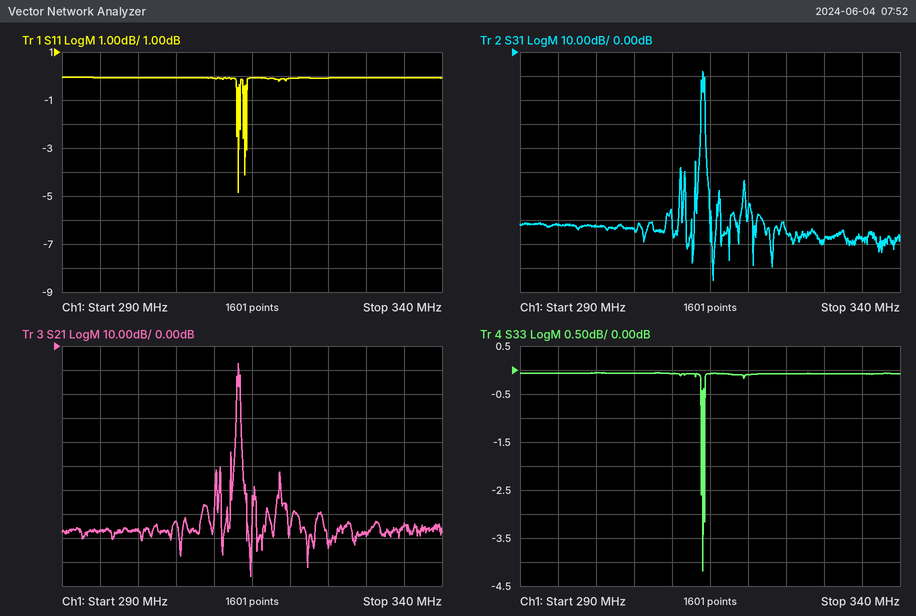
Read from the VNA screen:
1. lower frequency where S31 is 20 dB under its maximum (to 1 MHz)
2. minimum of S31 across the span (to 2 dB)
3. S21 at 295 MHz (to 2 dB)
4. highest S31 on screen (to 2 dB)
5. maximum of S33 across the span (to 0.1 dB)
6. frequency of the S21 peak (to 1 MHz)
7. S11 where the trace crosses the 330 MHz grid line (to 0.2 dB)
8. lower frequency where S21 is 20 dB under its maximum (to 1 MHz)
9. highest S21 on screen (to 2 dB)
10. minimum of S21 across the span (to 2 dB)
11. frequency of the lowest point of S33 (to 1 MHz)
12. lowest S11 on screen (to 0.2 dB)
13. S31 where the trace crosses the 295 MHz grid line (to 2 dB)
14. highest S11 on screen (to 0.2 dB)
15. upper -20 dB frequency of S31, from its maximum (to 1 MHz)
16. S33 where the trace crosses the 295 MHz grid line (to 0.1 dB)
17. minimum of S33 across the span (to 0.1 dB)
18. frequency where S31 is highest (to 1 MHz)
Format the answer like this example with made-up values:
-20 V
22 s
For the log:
314 MHz
-96 dB
-76 dB
-8 dB
-0.1 dB
313 MHz
0.0 dB
313 MHz
-8 dB
-96 dB
314 MHz
-4.8 dB
-72 dB
0.0 dB
314 MHz
-0.1 dB
-4.2 dB
314 MHz
